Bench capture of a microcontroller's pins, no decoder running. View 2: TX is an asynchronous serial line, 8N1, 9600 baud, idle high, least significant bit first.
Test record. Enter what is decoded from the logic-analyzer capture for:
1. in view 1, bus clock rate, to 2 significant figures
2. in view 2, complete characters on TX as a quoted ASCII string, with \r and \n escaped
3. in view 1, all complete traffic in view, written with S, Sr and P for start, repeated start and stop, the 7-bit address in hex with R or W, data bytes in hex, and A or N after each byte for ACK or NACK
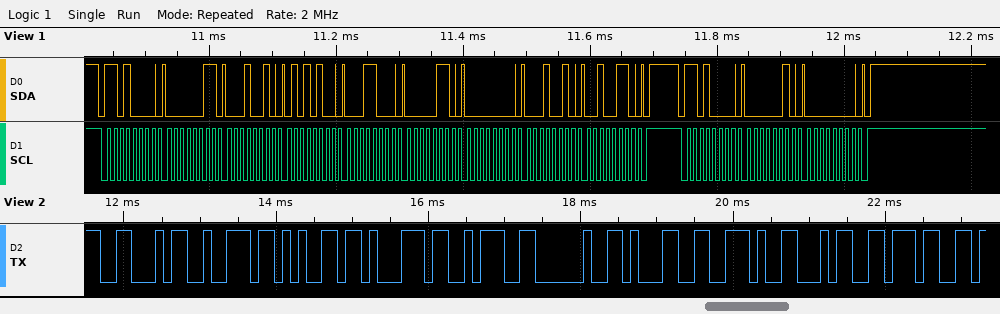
100 kHz
"Freq: 1.47"
S 68W A 03 A 12 A 54 A 18 A 06 A 00 A 12 A 26 A P S 68W A 02 A 00 A P
